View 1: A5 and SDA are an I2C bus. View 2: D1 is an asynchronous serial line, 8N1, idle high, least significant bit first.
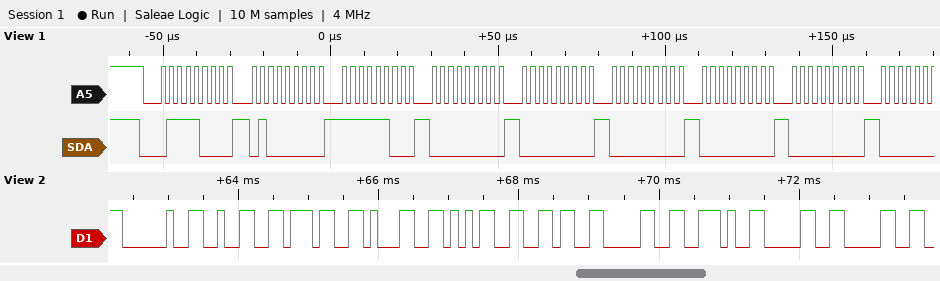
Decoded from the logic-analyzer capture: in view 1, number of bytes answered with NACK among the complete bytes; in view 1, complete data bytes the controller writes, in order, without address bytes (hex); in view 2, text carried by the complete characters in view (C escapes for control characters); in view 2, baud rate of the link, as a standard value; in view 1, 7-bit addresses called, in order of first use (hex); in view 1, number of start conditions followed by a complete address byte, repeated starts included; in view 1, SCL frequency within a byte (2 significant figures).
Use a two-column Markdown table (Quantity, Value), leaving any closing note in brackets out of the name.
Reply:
| Quantity | Value |
|---|---|
| in view 1, number of bytes answered with NACK among the complete bytes | 0 |
| in view 1, complete data bytes the controller writes, in order, without address bytes | 40 FC 00 00 00 00 00 |
| in view 2, text carried by the complete characters in view | " 271560.00" |
| in view 2, baud rate of the link, as a standard value | 9600 baud |
| in view 1, 7-bit addresses called, in order of first use | 0x3C |
| in view 1, number of start conditions followed by a complete address byte, repeated starts included | 1 |
| in view 1, SCL frequency within a byte | 400 kHz |
